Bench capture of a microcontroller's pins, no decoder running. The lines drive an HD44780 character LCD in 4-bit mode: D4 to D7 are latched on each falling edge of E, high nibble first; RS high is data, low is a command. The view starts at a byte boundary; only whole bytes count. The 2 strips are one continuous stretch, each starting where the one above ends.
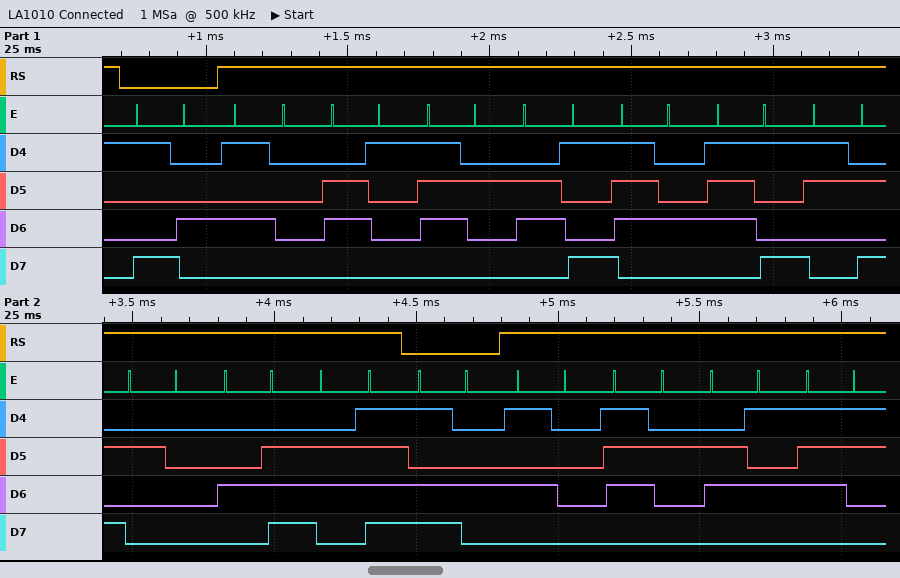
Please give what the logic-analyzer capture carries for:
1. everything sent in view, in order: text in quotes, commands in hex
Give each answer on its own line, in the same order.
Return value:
0x94 "Parity: No" 0xD4 "Pres"
